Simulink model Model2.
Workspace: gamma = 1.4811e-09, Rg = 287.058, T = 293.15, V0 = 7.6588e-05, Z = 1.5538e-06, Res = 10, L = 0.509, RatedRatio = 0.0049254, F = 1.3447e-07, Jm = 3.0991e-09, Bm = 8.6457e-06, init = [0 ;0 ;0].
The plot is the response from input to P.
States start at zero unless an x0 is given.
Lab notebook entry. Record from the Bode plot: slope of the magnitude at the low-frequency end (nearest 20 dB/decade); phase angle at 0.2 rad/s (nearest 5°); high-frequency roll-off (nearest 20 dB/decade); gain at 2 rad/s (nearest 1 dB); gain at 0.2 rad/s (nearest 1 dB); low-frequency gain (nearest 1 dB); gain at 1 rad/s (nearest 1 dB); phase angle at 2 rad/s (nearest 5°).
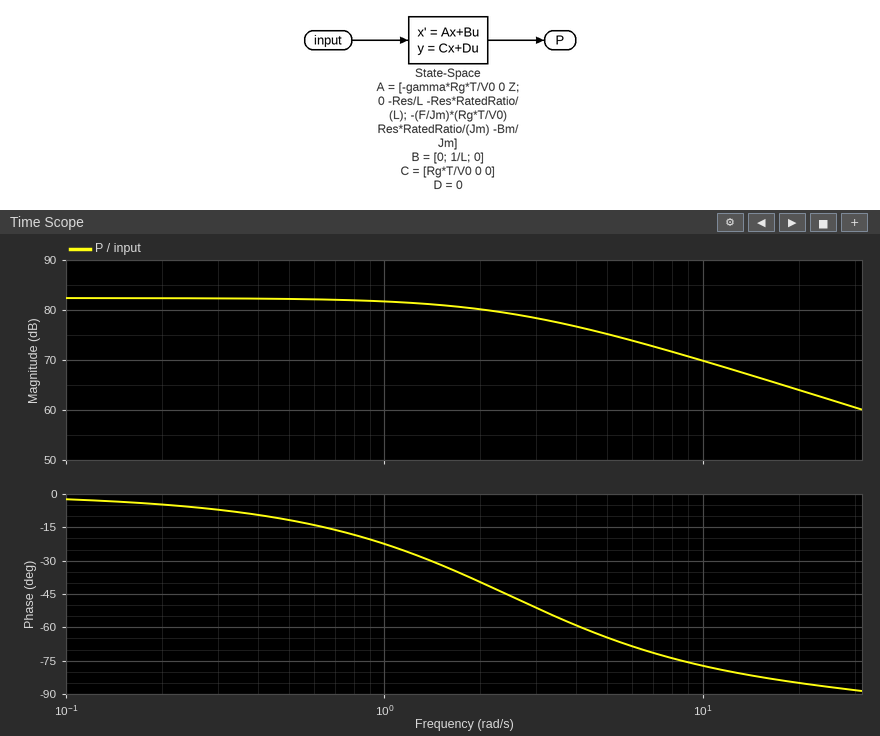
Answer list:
0 dB/decade
-5°
-20 dB/decade
80 dB
82 dB
82 dB
82 dB
-40°
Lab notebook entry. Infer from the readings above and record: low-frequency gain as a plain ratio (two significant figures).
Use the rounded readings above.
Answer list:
13000
